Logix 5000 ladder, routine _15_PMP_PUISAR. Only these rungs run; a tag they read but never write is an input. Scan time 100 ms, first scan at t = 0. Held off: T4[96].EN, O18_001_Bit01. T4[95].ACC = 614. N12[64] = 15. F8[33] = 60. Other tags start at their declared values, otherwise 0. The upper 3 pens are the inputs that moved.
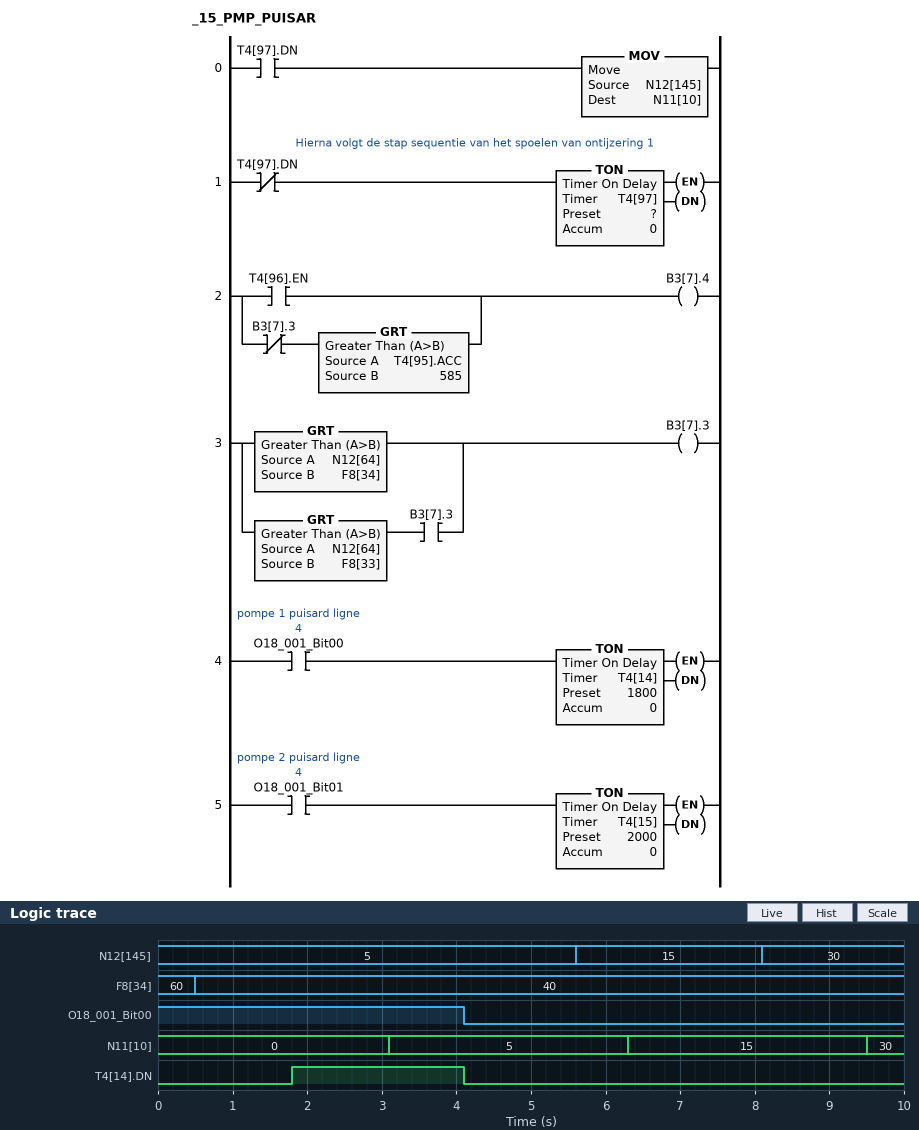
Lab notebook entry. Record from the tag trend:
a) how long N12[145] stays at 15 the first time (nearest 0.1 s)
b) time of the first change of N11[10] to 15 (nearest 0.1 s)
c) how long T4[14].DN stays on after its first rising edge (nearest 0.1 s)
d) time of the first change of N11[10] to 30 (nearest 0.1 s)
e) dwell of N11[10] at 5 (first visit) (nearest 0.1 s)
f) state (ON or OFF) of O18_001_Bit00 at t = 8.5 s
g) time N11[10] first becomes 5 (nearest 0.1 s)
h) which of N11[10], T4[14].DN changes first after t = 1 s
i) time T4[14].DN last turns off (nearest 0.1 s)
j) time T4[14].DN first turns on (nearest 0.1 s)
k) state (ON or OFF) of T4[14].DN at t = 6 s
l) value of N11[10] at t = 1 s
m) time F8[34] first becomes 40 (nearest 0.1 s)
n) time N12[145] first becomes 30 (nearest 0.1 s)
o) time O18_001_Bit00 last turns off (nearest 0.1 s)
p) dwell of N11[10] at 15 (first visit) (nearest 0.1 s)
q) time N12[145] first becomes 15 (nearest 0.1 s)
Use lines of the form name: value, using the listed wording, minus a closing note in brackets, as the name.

how long N12[145] stays at 15 the first time: 2.5 s
time of the first change of N11[10] to 15: 6.3 s
how long T4[14].DN stays on after its first rising edge: 2.3 s
time of the first change of N11[10] to 30: 9.5 s
dwell of N11[10] at 5 (first visit): 3.2 s
state (ON or OFF) of O18_001_Bit00 at t = 8.5 s: OFF
time N11[10] first becomes 5: 3.1 s
which of N11[10], T4[14].DN changes first after t = 1 s: T4[14].DN
time T4[14].DN last turns off: 4.1 s
time T4[14].DN first turns on: 1.8 s
state (ON or OFF) of T4[14].DN at t = 6 s: OFF
value of N11[10] at t = 1 s: 0
time F8[34] first becomes 40: 0.5 s
time N12[145] first becomes 30: 8.1 s
time O18_001_Bit00 last turns off: 4.1 s
dwell of N11[10] at 15 (first visit): 3.2 s
time N12[145] first becomes 15: 5.6 s
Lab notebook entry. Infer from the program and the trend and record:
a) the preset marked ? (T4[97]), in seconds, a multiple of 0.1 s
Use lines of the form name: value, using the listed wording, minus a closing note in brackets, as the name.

the preset marked ? (T4[97]), in seconds, a multiple of 0.1 s: 3.0 s
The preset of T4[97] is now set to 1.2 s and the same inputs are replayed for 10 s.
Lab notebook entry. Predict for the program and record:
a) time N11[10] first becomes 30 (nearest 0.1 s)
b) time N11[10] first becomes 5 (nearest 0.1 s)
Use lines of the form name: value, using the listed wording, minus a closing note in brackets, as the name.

time N11[10] first becomes 30: 8.3 s
time N11[10] first becomes 5: 1.3 s
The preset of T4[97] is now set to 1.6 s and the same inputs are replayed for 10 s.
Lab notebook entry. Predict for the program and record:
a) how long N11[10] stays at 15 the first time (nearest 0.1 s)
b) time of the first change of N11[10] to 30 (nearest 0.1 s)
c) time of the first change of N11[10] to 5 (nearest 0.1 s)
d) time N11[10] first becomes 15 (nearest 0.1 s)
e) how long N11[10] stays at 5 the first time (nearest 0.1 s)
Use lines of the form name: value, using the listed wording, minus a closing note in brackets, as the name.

how long N11[10] stays at 15 the first time: 1.8 s
time of the first change of N11[10] to 30: 8.9 s
time of the first change of N11[10] to 5: 1.7 s
time N11[10] first becomes 15: 7.1 s
how long N11[10] stays at 5 the first time: 5.4 s
